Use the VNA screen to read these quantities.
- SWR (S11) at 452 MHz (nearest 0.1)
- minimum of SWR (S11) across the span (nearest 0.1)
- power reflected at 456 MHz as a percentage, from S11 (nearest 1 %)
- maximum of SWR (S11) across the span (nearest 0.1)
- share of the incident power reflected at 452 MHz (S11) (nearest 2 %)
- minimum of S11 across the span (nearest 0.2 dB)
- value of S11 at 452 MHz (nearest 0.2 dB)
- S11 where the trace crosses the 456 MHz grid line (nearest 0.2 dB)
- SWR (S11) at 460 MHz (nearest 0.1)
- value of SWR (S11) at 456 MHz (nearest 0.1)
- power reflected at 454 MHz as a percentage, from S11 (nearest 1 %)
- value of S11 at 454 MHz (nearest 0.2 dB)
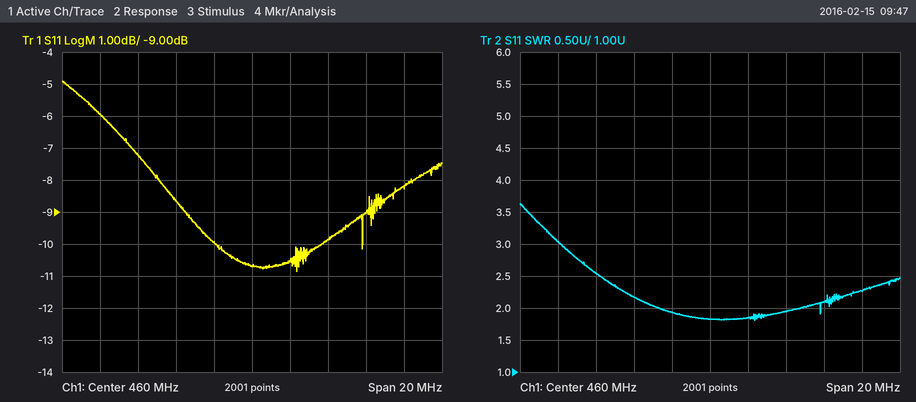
3.0
1.8
14 %
3.6
26 %
-10.8 dB
-6.0 dB
-8.6 dB
1.8
2.2
19 %
-7.2 dB
